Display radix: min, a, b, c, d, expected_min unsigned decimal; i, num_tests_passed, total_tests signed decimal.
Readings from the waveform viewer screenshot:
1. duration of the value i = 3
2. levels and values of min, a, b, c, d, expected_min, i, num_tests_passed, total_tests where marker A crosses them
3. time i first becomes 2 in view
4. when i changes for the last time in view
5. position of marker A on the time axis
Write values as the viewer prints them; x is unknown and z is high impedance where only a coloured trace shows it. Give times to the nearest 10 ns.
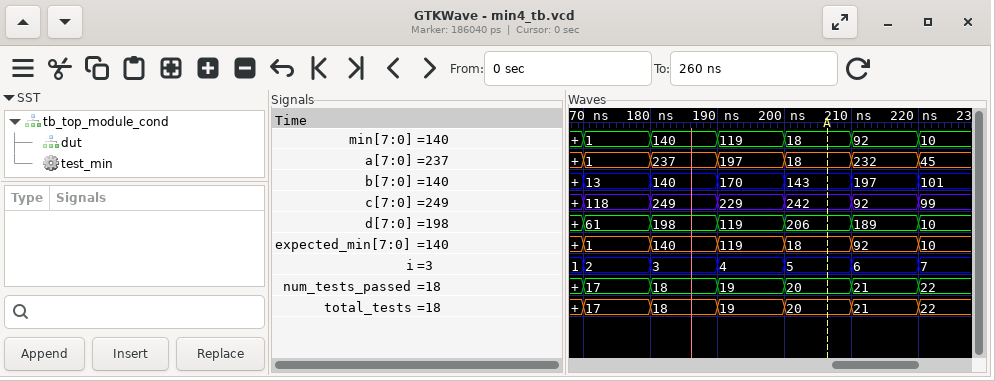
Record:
10 ns
min=18, a=18, b=143, c=242, d=206, expected_min=18, i=5, num_tests_passed=20, total_tests=20
170 ns
220 ns
210 ns
